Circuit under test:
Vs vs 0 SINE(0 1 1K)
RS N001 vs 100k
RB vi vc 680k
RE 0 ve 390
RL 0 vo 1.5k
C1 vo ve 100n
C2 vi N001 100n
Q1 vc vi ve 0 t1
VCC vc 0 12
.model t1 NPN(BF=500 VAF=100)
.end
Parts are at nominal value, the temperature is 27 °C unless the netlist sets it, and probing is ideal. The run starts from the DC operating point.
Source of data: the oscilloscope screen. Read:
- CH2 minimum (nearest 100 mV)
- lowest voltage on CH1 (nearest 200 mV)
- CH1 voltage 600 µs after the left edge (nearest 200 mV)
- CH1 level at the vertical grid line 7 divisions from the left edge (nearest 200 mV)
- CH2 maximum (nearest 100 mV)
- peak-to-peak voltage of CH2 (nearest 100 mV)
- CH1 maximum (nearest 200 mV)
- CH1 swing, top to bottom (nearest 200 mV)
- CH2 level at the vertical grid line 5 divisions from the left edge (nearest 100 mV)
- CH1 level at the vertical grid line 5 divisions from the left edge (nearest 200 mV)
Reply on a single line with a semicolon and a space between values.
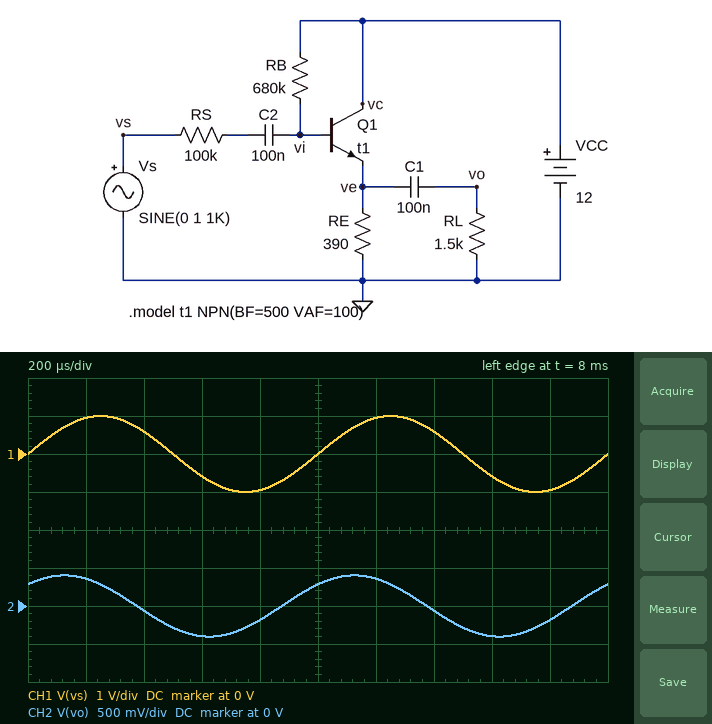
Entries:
-400 mV; -1.0 V; -600 mV; 600 mV; 400 mV; 800 mV; 1.0 V; 2.0 V; 300 mV; 0 V
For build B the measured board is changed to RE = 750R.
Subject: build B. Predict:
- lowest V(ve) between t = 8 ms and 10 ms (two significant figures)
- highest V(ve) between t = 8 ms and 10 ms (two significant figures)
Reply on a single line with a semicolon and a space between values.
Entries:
3.5 V; 4.8 V
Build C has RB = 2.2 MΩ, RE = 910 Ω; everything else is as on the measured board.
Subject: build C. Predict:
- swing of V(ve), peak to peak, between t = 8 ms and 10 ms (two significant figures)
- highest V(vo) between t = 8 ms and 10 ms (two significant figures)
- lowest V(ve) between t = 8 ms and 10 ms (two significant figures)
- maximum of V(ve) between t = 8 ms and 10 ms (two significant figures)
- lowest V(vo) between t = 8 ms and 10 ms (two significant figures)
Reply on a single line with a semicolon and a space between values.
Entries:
1.5 V; 520 mV; 1.3 V; 2.8 V; -520 mV
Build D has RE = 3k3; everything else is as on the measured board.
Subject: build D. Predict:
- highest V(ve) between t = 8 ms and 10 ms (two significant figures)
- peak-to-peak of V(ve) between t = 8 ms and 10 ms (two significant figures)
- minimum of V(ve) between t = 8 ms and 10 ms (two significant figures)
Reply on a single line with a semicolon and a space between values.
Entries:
8.8 V; 1.6 V; 7.2 V
